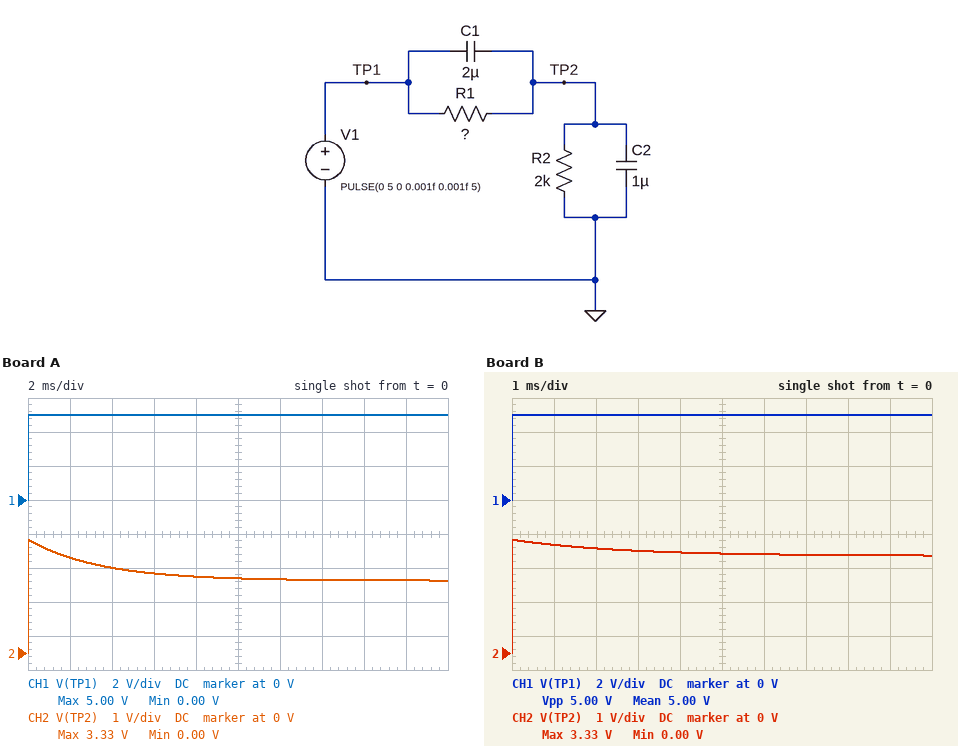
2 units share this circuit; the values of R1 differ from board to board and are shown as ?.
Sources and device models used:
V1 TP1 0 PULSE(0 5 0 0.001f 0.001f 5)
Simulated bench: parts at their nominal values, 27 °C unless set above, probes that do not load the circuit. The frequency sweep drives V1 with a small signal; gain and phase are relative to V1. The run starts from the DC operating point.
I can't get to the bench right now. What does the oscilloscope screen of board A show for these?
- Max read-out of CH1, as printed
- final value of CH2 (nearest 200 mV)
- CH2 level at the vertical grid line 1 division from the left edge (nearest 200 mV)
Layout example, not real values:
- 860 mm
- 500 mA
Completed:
- 5.00 V
- 2.2 V
- 2.8 V
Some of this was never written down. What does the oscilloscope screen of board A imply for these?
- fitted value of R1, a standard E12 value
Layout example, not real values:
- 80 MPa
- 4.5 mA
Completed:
- 2.7 kΩ
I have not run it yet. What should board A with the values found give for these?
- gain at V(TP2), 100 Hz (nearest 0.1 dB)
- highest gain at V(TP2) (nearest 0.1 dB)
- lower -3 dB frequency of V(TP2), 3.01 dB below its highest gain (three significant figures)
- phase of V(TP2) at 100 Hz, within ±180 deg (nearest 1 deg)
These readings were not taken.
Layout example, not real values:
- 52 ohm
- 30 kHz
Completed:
- -4.0 dB
- -3.5 dB
- 19.9 Hz
- 8 deg
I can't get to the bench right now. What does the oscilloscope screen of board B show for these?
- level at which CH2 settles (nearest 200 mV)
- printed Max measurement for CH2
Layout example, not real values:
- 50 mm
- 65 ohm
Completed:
- 2.8 V
- 3.33 V
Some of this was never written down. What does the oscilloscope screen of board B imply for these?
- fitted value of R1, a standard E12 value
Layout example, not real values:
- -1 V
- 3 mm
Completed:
- 1.5 kΩ
